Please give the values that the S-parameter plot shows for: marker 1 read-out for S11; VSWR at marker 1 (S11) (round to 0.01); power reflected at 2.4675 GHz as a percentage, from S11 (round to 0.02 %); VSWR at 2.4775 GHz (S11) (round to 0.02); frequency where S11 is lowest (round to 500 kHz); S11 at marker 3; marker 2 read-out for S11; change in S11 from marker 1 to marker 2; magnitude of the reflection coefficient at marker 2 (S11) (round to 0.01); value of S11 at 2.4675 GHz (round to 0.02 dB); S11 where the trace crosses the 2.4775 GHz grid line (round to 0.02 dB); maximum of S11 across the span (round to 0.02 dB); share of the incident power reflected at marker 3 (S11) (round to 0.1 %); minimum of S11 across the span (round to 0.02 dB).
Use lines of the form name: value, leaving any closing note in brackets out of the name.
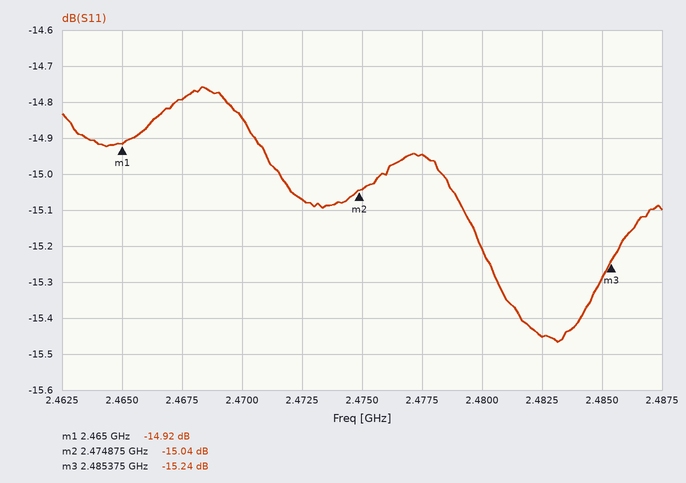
marker 1 read-out for S11: -14.92 dB
VSWR at marker 1 (S11): 1.44
power reflected at 2.4675 GHz as a percentage, from S11: 3.32 %
VSWR at 2.4775 GHz (S11): 1.44
frequency where S11 is lowest: 2.4830 GHz
S11 at marker 3: -15.24 dB
marker 2 read-out for S11: -15.04 dB
change in S11 from marker 1 to marker 2: -0.12 dB
magnitude of the reflection coefficient at marker 2 (S11): 0.18
value of S11 at 2.4675 GHz: -14.80 dB
S11 where the trace crosses the 2.4775 GHz grid line: -14.94 dB
maximum of S11 across the span: -14.76 dB
share of the incident power reflected at marker 3 (S11): 3.0 %
minimum of S11 across the span: -15.46 dB
